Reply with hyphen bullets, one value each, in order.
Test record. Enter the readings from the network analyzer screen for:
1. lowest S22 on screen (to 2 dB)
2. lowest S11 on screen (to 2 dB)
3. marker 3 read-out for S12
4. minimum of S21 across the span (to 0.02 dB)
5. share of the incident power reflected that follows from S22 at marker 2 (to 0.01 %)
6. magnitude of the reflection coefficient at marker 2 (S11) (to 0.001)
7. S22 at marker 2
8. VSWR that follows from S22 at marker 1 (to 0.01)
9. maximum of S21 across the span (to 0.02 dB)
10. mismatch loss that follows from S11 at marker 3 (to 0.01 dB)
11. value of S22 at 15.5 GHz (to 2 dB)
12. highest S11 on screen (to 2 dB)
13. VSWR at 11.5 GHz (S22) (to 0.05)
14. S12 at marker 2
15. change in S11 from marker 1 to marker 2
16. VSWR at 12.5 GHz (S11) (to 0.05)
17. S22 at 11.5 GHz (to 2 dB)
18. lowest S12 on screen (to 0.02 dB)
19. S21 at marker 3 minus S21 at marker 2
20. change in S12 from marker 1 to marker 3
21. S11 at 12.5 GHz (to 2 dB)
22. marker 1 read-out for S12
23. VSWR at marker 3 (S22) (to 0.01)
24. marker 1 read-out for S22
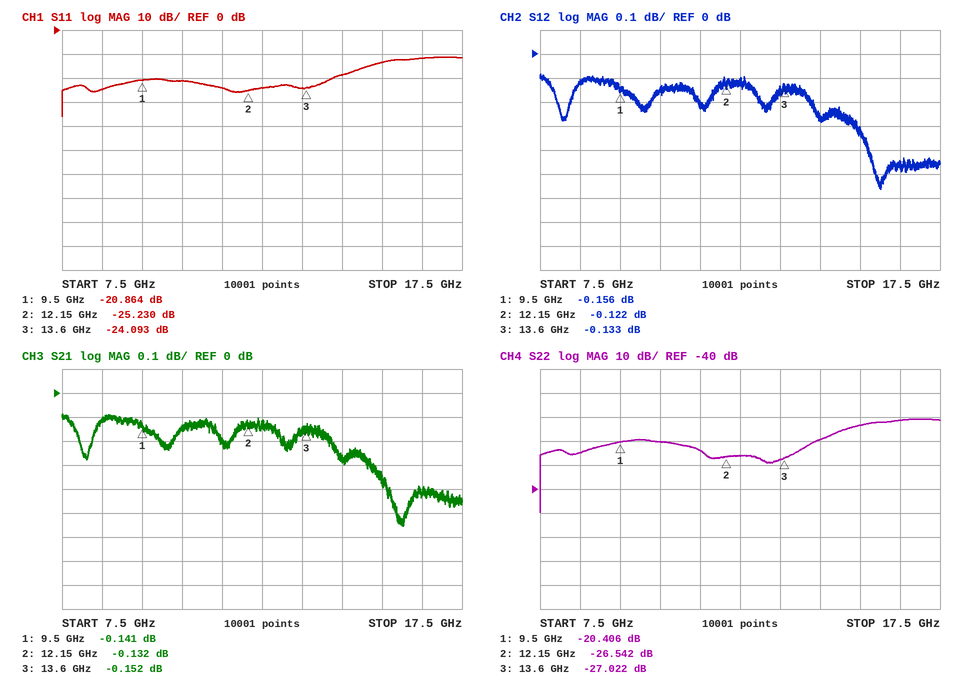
- -50 dB
- -36 dB
- -0.133 dB
- -0.56 dB
- 0.22 %
- 0.055
- -26.542 dB
- 1.21
- -0.08 dB
- 0.02 dB
- -14 dB
- -12 dB
- 1.15
- -0.122 dB
- -4.366 dB
- 1.15
- -24 dB
- -0.56 dB
- -0.020 dB
- 0.023 dB
- -24 dB
- -0.156 dB
- 1.09
- -20.406 dB
